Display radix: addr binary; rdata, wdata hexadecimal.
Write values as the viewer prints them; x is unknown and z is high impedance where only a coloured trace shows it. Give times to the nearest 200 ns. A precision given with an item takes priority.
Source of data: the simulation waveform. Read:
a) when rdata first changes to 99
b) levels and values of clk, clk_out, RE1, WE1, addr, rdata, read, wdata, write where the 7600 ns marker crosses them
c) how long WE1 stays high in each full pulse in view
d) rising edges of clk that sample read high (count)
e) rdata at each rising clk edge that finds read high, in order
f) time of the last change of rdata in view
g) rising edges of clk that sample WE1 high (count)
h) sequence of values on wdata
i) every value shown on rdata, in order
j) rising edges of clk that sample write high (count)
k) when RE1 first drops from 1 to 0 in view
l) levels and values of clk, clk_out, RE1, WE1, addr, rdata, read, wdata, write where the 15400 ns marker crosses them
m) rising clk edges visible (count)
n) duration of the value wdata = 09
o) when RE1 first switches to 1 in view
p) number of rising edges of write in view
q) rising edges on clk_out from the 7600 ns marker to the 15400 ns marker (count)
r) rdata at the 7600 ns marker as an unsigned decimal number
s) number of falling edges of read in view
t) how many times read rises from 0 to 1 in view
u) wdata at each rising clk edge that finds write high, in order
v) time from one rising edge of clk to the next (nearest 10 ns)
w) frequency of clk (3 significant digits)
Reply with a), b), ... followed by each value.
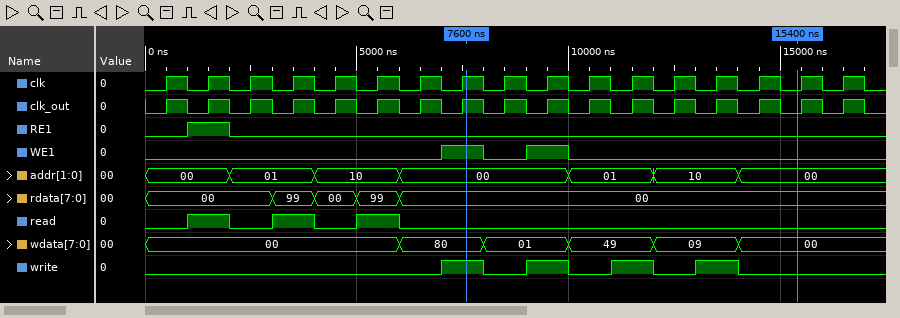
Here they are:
a) 3000 ns
b) clk=1, clk_out=1, RE1=0, WE1=1, addr=00, rdata=00, read=0, wdata=80, write=1
c) 1000 ns, 1000 ns
d) 3
e) 00, 99, 99
f) 6000 ns
g) 2
h) 00, 80, 01, 49, 09, 00
i) 00, 99, 00, 99, 00
j) 4
k) 2000 ns
l) clk=0, clk_out=0, RE1=0, WE1=0, addr=00, rdata=00, read=0, wdata=00, write=0
m) 17
n) 2000 ns
o) 1000 ns
p) 4
q) 7
r) 0
s) 3
t) 3
u) 80, 01, 49, 09
v) 1000 ns
w) 1.00 MHz
